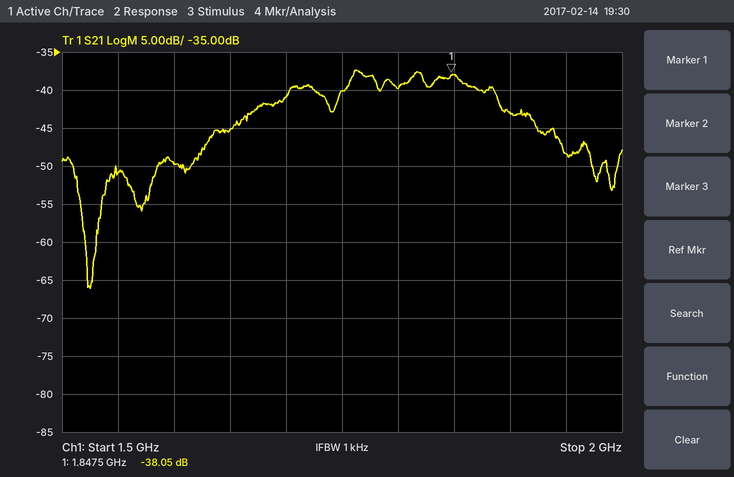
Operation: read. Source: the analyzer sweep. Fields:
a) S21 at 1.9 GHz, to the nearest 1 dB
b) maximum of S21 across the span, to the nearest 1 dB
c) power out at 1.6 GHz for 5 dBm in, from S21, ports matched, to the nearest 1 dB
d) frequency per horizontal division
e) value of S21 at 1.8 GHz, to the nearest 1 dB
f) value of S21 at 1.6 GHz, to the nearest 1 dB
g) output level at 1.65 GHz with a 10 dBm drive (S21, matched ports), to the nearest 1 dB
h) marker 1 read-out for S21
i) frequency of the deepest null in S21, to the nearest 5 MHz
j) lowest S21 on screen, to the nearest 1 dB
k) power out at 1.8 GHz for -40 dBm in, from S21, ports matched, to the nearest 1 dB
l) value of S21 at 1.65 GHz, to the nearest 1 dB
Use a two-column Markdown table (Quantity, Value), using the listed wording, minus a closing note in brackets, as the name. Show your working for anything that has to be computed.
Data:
| Quantity | Value |
|---|---|
| S21 at 1.9 GHz, to the nearest 1 dB | -43 dB |
| maximum of S21 across the span, to the nearest 1 dB | -37 dB |
| power out at 1.6 GHz for 5 dBm in, from S21, ports matched, to the nearest 1 dB | 5 dBm + (-50 dB) = -45 dBm |
| frequency per horizontal division | 50 MHz |
| value of S21 at 1.8 GHz, to the nearest 1 dB | -40 dB |
| value of S21 at 1.6 GHz, to the nearest 1 dB | -50 dB |
| output level at 1.65 GHz with a 10 dBm drive (S21, matched ports), to the nearest 1 dB | 10 dBm + (-45 dB) = -35 dBm |
| marker 1 read-out for S21 | -38.05 dB |
| frequency of the deepest null in S21, to the nearest 5 MHz | 1.525 GHz |
| lowest S21 on screen, to the nearest 1 dB | -66 dB |
| power out at 1.8 GHz for -40 dBm in, from S21, ports matched, to the nearest 1 dB | -40 dBm + (-40 dB) = -80 dBm |
| value of S21 at 1.65 GHz, to the nearest 1 dB | -45 dB |
